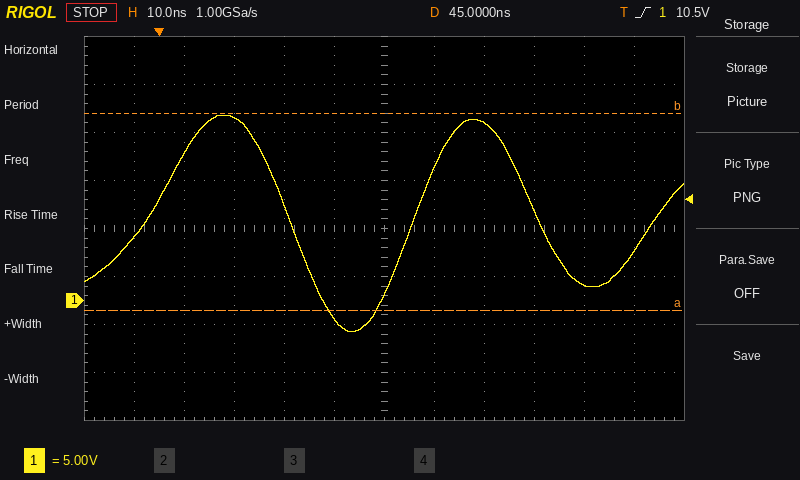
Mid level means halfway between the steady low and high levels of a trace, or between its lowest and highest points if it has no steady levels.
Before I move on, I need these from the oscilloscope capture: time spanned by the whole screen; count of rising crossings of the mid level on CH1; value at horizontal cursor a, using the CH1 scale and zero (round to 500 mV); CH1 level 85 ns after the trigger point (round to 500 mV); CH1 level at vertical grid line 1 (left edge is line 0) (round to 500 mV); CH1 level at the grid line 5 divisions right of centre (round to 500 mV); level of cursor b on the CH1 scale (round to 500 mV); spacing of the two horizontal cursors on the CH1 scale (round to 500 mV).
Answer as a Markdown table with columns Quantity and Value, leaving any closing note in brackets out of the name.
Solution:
| Quantity | Value |
|---|---|
| time spanned by the whole screen | 120 ns |
| count of rising crossings of the mid level on CH1 | 3 |
| value at horizontal cursor a, using the CH1 scale and zero | -1.0 V |
| CH1 level 85 ns after the trigger point | 1.5 V |
| CH1 level at vertical grid line 1 (left edge is line 0) | 6.5 V |
| CH1 level at the grid line 5 divisions right of centre | 5.0 V |
| level of cursor b on the CH1 scale | 19.5 V |
| spacing of the two horizontal cursors on the CH1 scale | 20.5 V |
